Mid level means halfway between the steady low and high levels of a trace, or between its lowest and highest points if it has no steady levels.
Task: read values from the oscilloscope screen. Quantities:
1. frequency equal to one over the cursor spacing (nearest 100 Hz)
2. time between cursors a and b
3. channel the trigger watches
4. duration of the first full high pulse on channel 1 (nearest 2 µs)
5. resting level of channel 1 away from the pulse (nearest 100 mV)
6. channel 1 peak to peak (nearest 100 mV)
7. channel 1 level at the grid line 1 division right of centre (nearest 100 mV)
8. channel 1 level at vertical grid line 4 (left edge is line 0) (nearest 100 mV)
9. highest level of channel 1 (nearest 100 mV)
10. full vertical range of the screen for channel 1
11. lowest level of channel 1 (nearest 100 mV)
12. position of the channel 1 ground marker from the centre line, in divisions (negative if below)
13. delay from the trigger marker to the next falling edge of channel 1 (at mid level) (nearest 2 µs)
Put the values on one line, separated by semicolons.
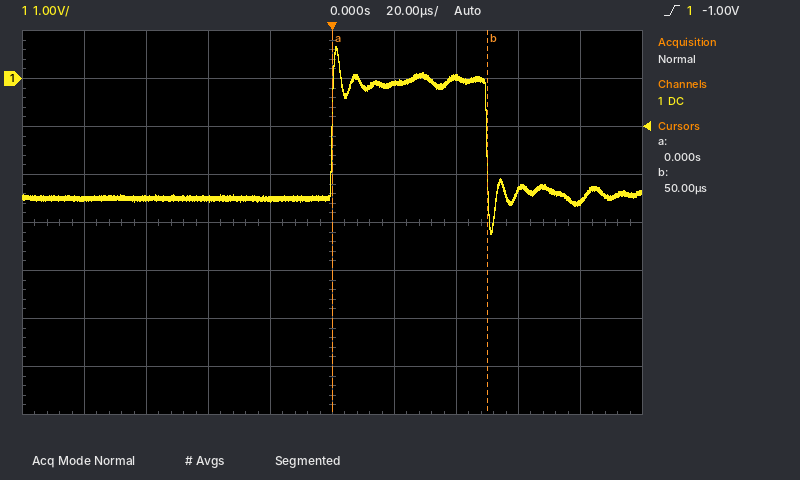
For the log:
20.0 kHz; 50 µs; channel 1; 50 µs; -2.5 V; 3.9 V; -100 mV; -2.5 V; 700 mV; 8 V; -3.2 V; +3.0 div; 50 µs
